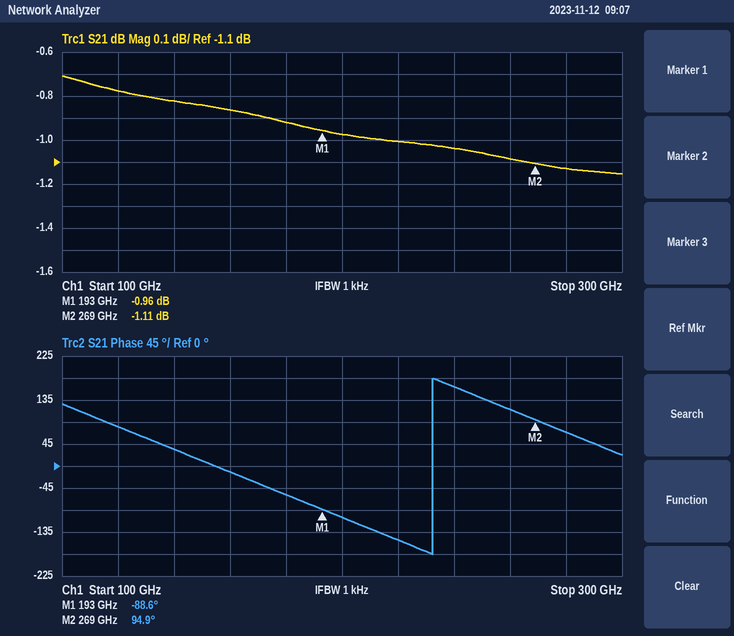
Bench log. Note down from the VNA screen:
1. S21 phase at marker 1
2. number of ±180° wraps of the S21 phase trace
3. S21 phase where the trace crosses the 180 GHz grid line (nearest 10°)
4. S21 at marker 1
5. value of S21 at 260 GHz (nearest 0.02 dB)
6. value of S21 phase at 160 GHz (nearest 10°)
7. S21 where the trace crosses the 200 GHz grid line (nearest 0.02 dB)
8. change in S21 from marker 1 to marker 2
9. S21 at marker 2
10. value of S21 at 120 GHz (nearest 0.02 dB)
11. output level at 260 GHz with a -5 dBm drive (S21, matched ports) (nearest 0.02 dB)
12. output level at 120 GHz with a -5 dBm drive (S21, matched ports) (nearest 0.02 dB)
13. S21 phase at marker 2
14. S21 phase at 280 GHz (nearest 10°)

-88.6°
1
-60°
-0.96 dB
-1.08 dB
-10°
-0.98 dB
-0.15 dB
-1.11 dB
-0.78 dB
-6.08 dBm
-5.78 dBm
94.9°
70°
